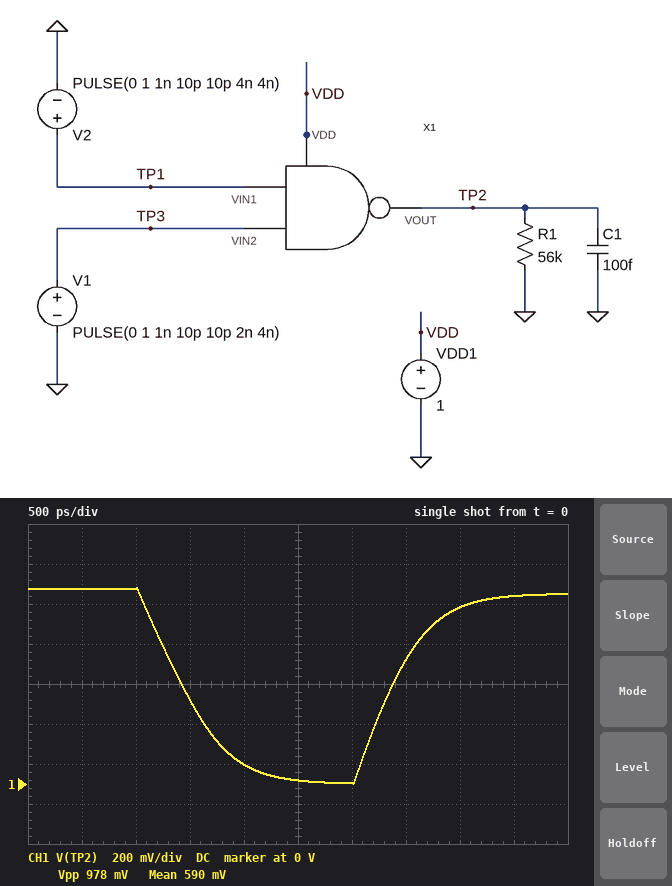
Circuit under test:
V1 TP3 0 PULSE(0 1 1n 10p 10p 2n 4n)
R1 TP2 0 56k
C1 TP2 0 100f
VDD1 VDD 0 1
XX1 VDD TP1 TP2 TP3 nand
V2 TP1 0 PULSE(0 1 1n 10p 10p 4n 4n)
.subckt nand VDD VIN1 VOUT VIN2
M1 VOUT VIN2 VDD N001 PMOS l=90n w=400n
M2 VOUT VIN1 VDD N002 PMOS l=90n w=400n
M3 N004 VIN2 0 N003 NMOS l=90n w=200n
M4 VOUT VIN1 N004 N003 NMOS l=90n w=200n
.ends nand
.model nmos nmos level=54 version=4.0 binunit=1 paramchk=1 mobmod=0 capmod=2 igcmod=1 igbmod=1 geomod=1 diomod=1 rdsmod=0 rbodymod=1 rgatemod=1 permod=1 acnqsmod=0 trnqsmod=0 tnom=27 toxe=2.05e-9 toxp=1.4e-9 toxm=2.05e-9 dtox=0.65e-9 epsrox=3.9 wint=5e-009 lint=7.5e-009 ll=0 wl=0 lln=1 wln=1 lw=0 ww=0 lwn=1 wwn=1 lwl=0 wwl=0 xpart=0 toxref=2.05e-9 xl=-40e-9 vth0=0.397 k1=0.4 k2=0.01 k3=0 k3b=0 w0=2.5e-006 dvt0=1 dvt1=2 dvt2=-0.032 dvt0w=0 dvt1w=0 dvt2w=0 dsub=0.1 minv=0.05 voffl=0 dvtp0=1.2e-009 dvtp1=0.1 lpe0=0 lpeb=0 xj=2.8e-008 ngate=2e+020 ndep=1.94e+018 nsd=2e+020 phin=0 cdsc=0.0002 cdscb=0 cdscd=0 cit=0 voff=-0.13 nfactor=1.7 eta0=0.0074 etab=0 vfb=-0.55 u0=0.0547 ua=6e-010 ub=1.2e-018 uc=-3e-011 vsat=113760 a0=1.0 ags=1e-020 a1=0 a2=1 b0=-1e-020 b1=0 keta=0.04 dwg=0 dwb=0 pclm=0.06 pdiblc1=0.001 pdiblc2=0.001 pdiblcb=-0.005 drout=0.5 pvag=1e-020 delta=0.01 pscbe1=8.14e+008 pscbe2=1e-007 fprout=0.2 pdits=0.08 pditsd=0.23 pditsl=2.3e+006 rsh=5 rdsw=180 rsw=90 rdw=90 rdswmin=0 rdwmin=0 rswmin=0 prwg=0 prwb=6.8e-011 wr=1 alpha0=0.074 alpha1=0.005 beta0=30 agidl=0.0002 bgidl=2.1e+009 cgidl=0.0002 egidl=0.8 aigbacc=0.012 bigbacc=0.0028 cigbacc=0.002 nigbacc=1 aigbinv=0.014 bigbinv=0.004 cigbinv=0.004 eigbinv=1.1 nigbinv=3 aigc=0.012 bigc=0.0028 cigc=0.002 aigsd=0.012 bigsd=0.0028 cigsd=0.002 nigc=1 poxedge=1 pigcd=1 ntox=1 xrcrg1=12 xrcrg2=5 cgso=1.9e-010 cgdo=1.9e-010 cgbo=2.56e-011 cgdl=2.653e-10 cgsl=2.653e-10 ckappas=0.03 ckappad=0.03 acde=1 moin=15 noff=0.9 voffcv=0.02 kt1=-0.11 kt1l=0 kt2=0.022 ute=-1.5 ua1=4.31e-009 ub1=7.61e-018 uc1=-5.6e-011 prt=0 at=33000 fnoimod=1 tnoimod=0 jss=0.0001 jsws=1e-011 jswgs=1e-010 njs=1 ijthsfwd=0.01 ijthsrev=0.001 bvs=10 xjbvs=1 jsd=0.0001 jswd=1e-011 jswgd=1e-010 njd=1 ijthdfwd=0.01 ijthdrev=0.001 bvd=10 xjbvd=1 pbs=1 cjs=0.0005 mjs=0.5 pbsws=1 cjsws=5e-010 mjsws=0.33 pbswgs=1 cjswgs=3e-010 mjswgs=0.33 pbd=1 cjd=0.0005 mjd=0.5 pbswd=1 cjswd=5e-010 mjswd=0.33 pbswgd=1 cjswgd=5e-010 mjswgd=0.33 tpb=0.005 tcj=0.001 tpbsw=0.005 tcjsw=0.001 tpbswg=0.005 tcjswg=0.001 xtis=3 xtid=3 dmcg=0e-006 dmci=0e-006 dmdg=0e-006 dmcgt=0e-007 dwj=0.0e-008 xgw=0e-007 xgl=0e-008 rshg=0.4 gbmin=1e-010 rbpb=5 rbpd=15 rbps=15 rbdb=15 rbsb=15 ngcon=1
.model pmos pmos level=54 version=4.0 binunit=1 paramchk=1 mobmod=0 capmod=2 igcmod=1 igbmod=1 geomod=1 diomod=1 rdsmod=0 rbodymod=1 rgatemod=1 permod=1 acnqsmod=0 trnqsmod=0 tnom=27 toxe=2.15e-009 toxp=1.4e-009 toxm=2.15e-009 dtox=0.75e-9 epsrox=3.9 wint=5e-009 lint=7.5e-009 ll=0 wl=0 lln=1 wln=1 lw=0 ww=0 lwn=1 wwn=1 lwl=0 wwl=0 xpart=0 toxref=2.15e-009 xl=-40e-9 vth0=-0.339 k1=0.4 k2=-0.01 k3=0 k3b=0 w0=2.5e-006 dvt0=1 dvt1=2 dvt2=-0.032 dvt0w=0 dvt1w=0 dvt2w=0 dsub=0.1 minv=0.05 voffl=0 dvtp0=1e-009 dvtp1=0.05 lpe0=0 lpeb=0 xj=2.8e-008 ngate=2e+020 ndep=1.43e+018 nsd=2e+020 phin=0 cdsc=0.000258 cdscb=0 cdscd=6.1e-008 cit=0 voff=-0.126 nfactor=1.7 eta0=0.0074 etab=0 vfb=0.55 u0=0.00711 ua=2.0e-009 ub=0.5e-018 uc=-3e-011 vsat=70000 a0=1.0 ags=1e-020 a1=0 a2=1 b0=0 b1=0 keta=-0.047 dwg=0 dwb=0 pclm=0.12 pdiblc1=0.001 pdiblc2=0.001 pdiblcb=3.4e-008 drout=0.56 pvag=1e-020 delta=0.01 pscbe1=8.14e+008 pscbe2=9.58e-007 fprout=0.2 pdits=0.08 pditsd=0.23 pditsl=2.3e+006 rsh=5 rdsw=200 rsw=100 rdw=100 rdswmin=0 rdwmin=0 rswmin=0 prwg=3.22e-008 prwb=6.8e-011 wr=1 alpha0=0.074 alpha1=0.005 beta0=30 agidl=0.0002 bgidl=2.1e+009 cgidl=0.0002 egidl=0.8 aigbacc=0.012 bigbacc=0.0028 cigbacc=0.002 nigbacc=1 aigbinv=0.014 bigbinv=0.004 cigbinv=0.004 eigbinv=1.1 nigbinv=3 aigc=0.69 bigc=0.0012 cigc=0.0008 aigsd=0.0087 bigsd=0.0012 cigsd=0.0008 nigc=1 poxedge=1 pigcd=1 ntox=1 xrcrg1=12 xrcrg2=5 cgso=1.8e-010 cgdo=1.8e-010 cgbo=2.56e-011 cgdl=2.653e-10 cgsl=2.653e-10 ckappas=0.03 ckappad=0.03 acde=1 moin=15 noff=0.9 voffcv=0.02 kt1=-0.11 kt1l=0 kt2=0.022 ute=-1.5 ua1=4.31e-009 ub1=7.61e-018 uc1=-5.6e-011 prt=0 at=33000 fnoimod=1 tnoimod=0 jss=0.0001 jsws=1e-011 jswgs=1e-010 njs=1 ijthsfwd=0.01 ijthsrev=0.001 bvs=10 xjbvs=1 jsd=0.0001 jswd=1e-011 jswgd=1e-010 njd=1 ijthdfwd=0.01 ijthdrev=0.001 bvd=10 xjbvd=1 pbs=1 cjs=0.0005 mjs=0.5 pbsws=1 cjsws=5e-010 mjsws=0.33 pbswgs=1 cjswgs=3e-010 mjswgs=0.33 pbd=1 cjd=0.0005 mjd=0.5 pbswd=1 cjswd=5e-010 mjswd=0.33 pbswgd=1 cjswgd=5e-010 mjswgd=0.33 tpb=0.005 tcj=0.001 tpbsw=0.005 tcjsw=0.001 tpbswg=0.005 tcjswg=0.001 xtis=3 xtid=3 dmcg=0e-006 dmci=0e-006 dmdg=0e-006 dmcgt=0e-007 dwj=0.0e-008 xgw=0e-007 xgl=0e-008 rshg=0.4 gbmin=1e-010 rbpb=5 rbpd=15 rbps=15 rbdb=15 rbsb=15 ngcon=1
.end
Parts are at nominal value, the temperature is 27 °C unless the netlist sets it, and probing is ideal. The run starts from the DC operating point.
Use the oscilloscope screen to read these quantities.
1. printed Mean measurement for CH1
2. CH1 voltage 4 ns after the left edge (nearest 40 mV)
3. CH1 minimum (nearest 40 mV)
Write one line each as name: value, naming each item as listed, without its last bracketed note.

printed Mean measurement for CH1: 590 mV
CH1 voltage 4 ns after the left edge: 880 mV
CH1 minimum: 0 V
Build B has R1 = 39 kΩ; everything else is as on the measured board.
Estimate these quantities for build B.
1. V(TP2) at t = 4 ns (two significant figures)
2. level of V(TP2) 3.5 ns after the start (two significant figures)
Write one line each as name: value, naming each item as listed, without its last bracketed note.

V(TP2) at t = 4 ns: 860 mV
level of V(TP2) 3.5 ns after the start: 610 mV
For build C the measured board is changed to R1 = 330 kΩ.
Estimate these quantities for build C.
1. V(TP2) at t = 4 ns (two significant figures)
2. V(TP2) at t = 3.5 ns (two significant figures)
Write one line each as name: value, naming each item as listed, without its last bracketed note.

V(TP2) at t = 4 ns: 920 mV
V(TP2) at t = 3.5 ns: 640 mV
